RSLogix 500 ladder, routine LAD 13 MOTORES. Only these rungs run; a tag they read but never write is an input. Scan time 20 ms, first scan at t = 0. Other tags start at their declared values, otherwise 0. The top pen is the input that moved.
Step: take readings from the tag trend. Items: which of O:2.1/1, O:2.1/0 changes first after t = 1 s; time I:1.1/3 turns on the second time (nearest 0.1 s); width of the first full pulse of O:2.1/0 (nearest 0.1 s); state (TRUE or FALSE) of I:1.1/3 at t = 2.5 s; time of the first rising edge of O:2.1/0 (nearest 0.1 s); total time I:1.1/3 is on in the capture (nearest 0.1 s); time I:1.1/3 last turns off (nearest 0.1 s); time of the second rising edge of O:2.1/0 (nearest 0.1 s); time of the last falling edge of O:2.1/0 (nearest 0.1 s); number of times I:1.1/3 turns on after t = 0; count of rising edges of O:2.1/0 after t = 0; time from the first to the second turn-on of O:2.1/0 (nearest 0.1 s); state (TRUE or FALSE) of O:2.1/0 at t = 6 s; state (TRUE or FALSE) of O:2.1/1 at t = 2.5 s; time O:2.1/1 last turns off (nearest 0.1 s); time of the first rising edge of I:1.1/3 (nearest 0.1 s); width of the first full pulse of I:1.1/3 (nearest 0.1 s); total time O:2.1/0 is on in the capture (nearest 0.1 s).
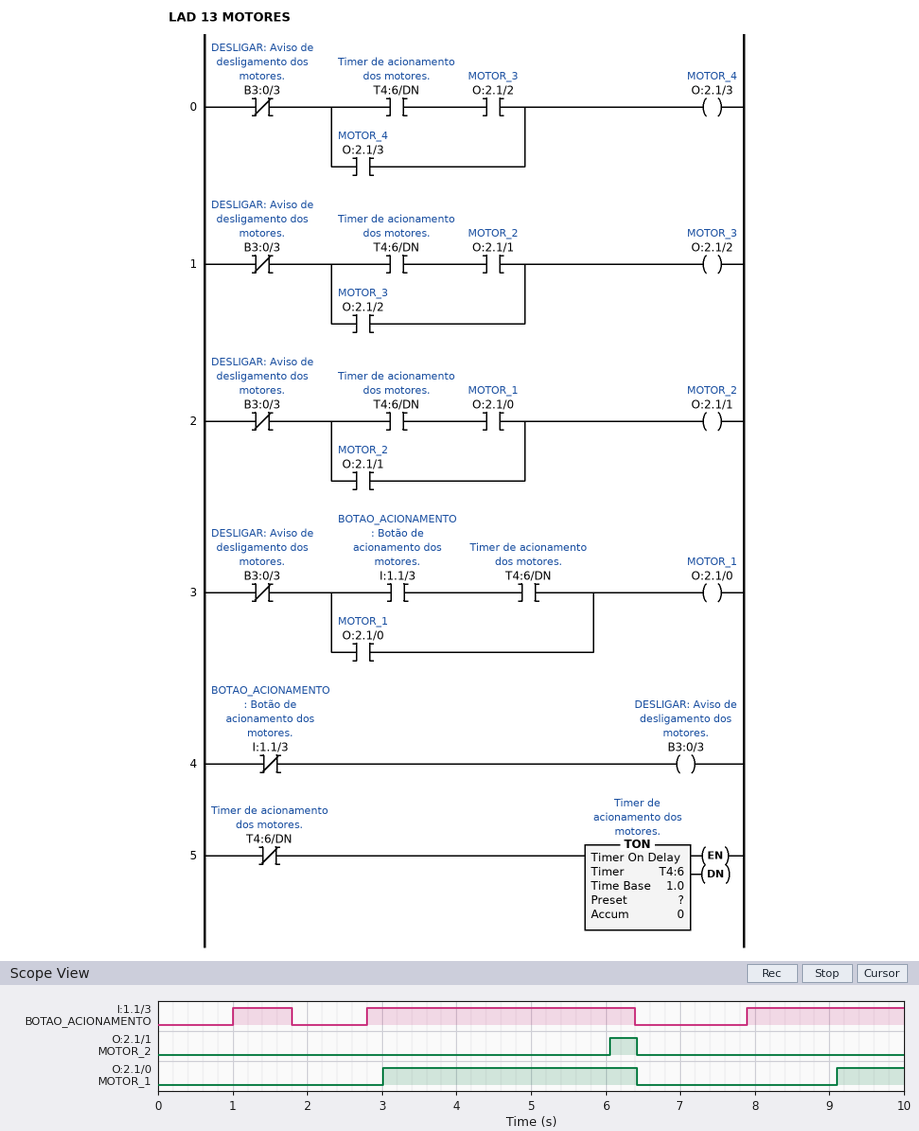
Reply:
O:2.1/0
2.8 s
3.4 s
FALSE
3.0 s
6.5 s
6.4 s
9.1 s
6.4 s
3
2
6.1 s
TRUE
FALSE
6.4 s
1.0 s
0.8 s
4.3 s
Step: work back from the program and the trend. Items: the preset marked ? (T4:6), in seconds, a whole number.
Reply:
3 s
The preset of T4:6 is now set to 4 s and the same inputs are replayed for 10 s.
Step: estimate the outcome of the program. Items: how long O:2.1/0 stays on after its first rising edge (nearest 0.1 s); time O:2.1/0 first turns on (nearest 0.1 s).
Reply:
2.4 s
4.0 s
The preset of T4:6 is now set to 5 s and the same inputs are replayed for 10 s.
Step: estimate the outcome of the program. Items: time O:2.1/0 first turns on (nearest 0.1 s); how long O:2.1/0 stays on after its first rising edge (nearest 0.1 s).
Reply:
5.0 s
1.4 s
